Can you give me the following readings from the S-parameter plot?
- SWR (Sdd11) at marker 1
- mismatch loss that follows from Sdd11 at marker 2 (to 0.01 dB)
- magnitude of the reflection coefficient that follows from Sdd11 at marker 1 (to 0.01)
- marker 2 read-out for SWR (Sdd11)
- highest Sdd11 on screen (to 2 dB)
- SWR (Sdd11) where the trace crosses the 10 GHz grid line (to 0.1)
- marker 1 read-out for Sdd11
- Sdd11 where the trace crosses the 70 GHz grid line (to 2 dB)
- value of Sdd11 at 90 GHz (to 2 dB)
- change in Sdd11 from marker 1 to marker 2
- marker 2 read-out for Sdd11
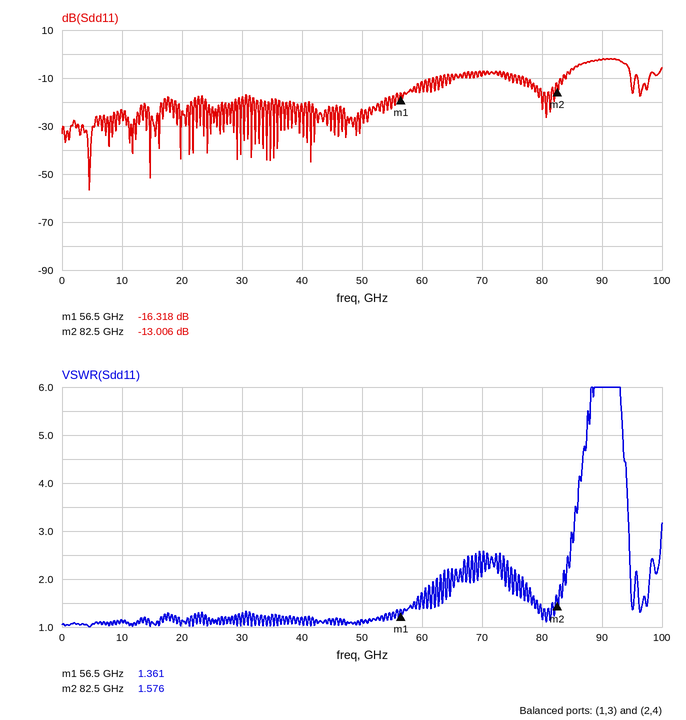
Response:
1.361
0.22 dB
0.15
1.576
-2 dB
1.1
-16.318 dB
-8 dB
-2 dB
3.312 dB
-13.006 dB
